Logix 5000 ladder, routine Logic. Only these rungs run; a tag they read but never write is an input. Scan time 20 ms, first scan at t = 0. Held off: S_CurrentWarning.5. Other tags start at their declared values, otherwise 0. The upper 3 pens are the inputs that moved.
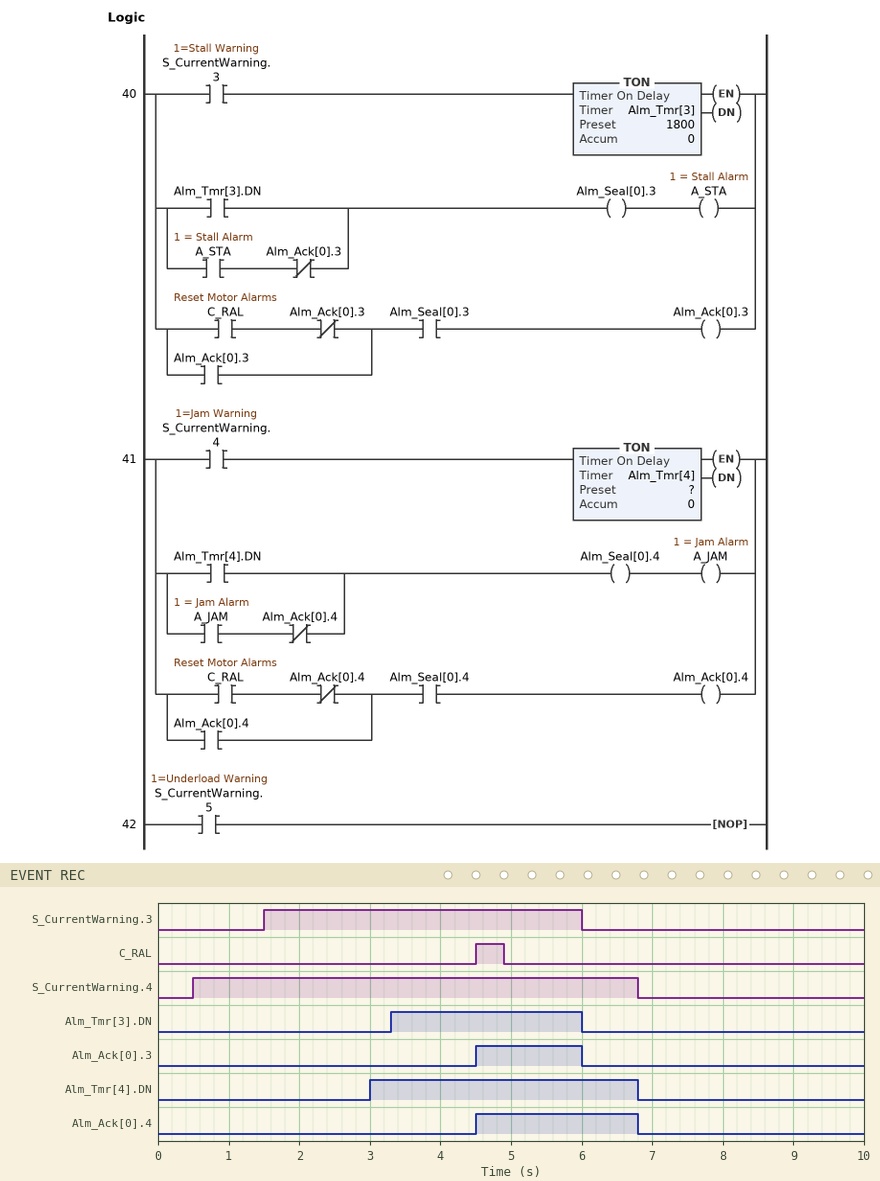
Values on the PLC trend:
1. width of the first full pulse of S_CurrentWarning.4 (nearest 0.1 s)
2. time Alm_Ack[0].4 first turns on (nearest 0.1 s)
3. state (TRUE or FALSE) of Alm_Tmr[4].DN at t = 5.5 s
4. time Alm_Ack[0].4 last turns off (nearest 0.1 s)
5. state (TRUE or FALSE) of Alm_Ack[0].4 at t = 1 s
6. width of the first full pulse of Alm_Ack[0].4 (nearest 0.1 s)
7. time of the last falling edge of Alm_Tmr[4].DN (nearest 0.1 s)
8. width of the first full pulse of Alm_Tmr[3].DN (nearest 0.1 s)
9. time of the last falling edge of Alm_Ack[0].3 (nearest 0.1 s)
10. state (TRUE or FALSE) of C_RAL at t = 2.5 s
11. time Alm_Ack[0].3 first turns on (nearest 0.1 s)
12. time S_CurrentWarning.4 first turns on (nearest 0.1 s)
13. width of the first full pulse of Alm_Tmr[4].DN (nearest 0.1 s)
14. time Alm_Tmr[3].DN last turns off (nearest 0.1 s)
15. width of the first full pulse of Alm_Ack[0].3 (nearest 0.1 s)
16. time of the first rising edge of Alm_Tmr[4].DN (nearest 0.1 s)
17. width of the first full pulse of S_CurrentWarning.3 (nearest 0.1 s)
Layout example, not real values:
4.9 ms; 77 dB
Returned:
6.3 s; 4.5 s; TRUE; 6.8 s; FALSE; 2.3 s; 6.8 s; 2.7 s; 6.0 s; FALSE; 4.5 s; 0.5 s; 3.8 s; 6.0 s; 1.5 s; 3.0 s; 4.5 s
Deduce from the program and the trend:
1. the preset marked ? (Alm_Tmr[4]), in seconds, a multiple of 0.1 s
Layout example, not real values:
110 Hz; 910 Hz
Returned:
2.5 s
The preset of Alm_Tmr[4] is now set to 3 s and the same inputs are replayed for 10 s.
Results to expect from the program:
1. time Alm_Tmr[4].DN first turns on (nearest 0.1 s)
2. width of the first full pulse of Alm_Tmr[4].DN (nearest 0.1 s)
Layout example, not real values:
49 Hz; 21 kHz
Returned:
3.5 s; 3.3 s
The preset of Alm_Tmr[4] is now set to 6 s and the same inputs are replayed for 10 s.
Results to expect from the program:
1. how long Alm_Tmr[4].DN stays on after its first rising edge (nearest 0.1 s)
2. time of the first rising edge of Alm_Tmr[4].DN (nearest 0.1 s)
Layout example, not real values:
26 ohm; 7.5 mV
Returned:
0.3 s; 6.5 s
